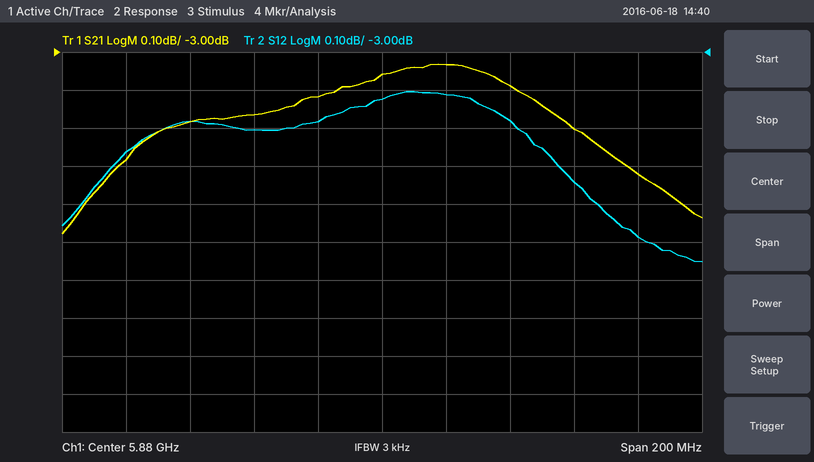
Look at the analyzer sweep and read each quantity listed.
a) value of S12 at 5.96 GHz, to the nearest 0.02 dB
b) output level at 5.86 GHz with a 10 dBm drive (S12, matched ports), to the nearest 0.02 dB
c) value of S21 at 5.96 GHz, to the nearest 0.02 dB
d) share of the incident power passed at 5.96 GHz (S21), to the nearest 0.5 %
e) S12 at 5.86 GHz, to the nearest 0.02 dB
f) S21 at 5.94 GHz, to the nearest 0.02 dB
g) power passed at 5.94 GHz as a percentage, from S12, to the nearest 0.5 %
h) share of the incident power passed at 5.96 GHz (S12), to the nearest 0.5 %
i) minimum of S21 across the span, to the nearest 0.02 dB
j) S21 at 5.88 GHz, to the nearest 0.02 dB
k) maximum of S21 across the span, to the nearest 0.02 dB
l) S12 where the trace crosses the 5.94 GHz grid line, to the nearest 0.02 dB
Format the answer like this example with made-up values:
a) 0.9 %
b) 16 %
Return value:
a) -3.48 dB
b) 6.82 dBm
c) -3.32 dB
d) 46.5 %
e) -3.18 dB
f) -3.20 dB
g) 46.5 %
h) 45.0 %
i) -3.48 dB
j) -3.06 dB
k) -3.04 dB
l) -3.34 dB
